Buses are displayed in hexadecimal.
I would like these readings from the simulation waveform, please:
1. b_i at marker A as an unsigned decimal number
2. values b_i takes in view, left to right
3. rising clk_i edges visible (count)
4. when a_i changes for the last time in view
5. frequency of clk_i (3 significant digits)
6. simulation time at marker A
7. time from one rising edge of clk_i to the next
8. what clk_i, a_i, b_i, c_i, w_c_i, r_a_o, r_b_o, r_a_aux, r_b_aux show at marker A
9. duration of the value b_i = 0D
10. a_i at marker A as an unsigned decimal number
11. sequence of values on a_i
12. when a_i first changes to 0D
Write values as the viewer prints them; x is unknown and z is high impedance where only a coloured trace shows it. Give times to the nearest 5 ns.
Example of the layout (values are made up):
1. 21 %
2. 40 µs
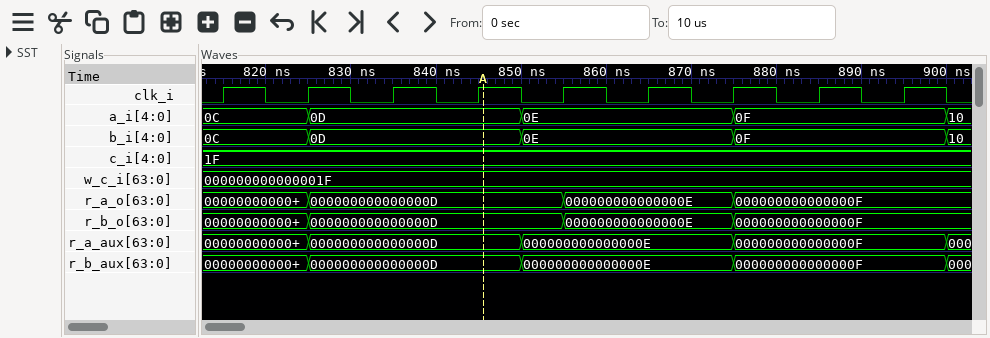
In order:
1. 13
2. 0C, 0D, 0E, 0F, 10
3. 9
4. 900 ns
5. 100 MHz
6. 845 ns
7. 10 ns
8. clk_i=1, a_i=0D, b_i=0D, c_i=1F, w_c_i=000000000000001F, r_a_o=000000000000000D, r_b_o=000000000000000D, r_a_aux=000000000000000D, r_b_aux=000000000000000D
9. 25 ns
10. 13
11. 0C, 0D, 0E, 0F, 10
12. 825 ns
